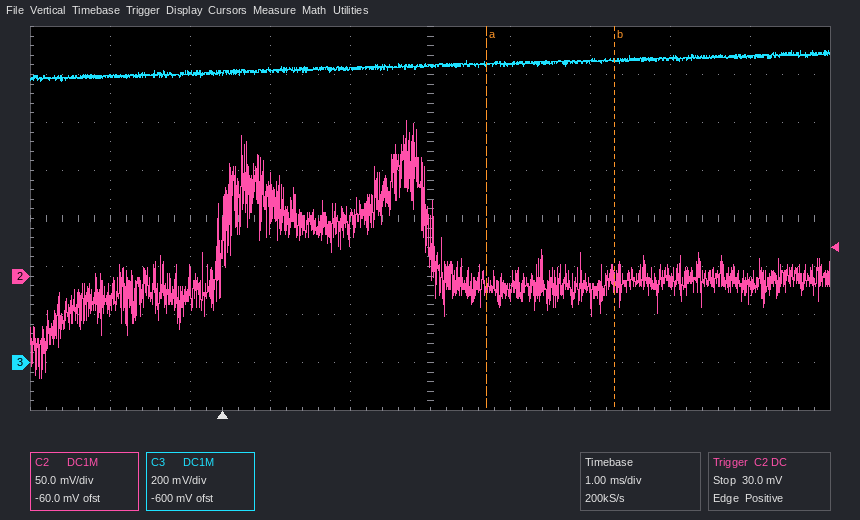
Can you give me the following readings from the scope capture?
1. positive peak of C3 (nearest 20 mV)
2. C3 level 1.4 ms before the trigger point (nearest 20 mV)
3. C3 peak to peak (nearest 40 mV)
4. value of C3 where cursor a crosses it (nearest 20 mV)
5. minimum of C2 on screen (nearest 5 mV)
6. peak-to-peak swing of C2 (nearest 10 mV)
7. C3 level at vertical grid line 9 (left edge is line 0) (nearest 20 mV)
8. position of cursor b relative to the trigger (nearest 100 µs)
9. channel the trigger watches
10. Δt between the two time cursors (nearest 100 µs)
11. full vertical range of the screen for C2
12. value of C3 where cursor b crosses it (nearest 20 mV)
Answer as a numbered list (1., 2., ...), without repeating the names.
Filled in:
1. 1.30 V
2. 1.20 V
3. 120 mV
4. 1.24 V
5. -105 mV
6. 270 mV
7. 1.28 V
8. +4.9 ms
9. C2
10. 1.6 ms
11. 400 mV
12. 1.26 V
